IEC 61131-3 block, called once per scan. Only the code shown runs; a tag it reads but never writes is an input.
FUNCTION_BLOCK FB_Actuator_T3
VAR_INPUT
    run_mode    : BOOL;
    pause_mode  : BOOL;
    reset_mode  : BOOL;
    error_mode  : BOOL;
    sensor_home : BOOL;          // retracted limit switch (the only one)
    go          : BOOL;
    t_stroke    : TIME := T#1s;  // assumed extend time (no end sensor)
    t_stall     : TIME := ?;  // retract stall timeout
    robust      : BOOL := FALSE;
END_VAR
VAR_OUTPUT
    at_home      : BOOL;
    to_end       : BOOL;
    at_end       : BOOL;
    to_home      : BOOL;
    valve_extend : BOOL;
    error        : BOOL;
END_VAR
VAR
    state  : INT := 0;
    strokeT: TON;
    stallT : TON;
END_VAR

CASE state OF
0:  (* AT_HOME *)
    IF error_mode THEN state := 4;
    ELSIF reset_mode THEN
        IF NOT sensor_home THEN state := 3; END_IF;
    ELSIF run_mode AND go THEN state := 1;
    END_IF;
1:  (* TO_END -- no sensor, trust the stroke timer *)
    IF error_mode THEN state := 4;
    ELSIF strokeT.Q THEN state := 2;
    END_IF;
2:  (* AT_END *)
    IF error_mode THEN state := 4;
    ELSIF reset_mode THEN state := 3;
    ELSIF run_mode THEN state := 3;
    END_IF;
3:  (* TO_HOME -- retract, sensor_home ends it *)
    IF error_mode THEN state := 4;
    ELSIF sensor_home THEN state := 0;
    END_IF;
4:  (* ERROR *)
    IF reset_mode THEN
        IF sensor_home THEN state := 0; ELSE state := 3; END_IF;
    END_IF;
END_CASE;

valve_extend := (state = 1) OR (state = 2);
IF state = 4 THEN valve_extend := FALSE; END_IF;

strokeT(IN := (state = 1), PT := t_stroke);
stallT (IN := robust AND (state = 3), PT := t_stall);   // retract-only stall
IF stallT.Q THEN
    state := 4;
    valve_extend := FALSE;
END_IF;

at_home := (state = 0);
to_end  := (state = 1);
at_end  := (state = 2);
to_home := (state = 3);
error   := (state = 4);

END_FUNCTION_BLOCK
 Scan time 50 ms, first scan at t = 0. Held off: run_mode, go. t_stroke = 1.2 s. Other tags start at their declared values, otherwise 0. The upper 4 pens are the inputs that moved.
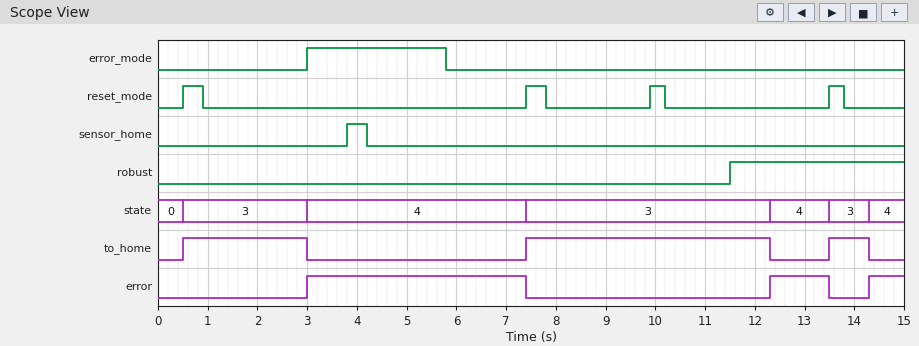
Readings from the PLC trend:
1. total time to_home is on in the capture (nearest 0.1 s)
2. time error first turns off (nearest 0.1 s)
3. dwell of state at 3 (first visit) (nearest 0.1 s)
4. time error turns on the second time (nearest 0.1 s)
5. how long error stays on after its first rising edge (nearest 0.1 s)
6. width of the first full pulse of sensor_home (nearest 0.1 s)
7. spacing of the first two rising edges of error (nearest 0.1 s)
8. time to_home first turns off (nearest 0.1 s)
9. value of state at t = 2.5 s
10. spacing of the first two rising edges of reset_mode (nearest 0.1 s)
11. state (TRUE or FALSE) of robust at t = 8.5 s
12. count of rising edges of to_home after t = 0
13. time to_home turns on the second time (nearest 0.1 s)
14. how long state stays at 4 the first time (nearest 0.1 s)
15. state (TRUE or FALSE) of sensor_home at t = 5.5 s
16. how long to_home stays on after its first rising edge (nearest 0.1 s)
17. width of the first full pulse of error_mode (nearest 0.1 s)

8.2 s
7.4 s
2.5 s
12.3 s
4.4 s
0.4 s
9.3 s
3.0 s
3
6.9 s
FALSE
3
7.4 s
4.4 s
FALSE
2.5 s
2.8 s
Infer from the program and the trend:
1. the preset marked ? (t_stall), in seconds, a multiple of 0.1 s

0.8 s
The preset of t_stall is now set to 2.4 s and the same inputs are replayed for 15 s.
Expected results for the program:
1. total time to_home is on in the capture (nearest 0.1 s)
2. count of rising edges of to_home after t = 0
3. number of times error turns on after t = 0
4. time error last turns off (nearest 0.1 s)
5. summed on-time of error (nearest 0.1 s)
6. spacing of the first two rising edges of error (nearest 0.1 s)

9.0 s
2
2
7.4 s
5.5 s
10.9 s
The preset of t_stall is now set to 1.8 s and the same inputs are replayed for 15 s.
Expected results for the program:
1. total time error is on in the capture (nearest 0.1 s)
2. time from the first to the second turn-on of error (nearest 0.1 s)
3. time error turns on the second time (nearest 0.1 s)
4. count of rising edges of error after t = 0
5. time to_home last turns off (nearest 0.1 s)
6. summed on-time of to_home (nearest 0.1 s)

4.6 s
10.3 s
13.3 s
2
13.3 s
9.9 s
